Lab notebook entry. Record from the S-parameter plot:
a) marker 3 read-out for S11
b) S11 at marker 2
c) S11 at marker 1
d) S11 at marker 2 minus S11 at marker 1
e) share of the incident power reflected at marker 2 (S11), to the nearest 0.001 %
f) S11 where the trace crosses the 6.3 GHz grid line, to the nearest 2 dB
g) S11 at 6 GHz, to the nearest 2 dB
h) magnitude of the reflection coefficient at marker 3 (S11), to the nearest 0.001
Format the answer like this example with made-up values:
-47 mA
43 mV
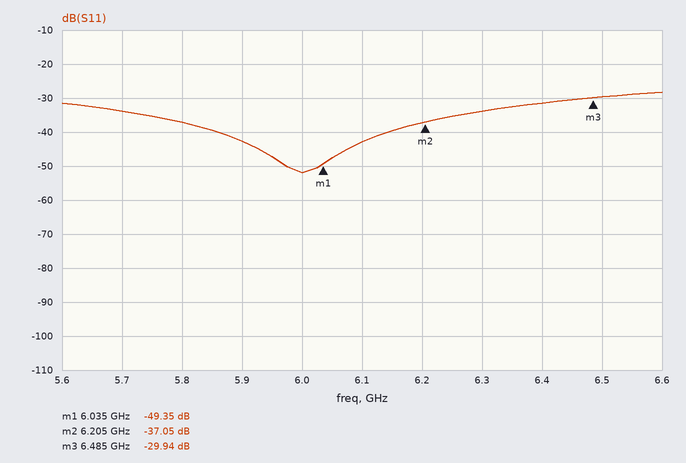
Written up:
-29.94 dB
-37.05 dB
-49.35 dB
12.30 dB
0.020 %
-34 dB
-52 dB
0.032
